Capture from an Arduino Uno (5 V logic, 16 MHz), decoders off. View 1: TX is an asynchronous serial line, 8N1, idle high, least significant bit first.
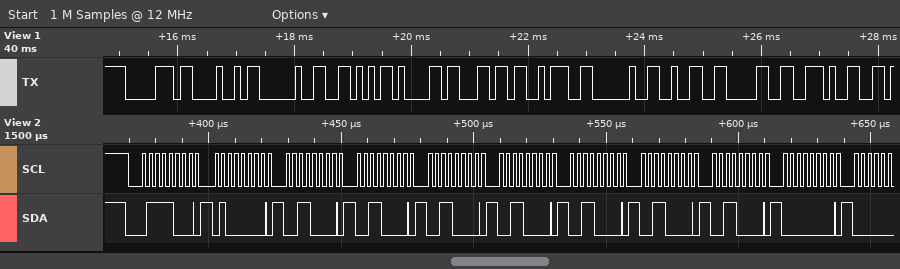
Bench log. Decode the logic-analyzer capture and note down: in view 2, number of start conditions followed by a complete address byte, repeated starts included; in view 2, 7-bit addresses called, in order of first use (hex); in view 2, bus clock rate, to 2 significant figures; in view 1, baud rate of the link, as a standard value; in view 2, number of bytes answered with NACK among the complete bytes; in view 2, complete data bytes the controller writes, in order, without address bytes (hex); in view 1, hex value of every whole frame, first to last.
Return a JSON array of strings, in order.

["1", "0x3C", "400 kHz", "9600 baud", "0", "40 30 30 30 30 30 30 30 00", "0x70 0x48 0x20 0x56 0x61 0x6C 0x3A 0x20 0x32 0x30 0x2E"]
